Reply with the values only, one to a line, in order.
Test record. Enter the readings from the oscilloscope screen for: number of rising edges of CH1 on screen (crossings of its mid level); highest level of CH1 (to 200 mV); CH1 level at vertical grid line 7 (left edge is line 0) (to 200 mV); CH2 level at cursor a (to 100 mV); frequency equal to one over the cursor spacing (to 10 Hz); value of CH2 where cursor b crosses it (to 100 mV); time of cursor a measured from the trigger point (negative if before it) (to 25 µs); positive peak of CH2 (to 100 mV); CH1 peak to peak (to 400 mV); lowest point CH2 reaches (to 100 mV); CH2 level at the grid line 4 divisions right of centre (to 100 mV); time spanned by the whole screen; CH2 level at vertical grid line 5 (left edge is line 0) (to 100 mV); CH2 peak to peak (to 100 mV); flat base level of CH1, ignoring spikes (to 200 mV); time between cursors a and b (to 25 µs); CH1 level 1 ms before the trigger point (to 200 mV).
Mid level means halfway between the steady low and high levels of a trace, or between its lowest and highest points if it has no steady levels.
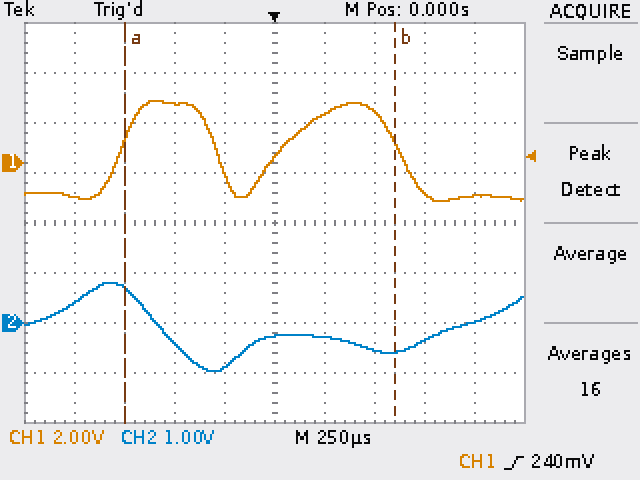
2
2.4 V
2.0 V
700 mV
740 Hz
-600 mV
-750 µs
800 mV
4.0 V
-1.0 V
0.0 V
2.5 ms
-300 mV
1.8 V
-1.4 V
1.350 ms
-1.4 V
